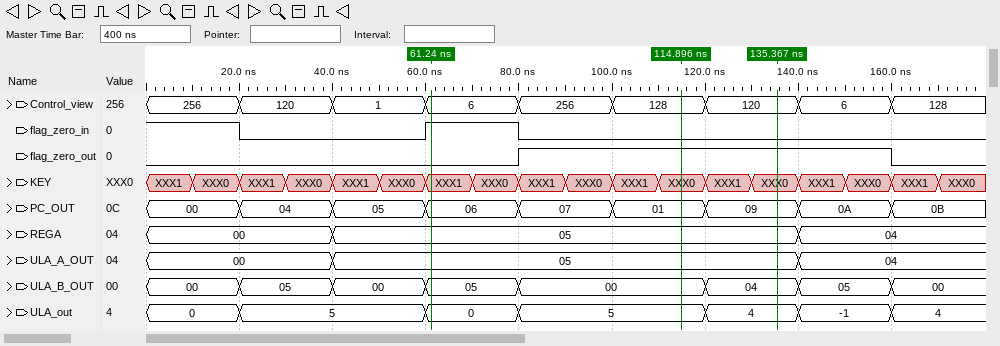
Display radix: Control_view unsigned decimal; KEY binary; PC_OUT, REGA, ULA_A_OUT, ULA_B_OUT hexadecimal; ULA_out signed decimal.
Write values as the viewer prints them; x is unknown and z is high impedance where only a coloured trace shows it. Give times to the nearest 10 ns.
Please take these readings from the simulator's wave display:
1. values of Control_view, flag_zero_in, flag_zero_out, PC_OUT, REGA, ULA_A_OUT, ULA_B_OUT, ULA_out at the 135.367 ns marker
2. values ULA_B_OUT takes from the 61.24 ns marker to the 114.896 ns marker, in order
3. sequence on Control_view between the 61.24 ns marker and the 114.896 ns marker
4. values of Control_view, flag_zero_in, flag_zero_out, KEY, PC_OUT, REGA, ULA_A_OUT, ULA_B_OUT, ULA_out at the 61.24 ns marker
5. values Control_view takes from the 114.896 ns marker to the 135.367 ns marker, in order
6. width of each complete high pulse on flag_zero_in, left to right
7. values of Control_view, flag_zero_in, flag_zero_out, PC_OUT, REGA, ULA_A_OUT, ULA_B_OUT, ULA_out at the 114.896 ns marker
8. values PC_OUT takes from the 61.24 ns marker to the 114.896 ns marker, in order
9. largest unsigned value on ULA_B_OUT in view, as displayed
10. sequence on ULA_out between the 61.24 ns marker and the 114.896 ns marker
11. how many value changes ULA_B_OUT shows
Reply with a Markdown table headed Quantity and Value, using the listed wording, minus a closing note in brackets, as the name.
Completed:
| Quantity | Value |
|---|---|
| values of Control_view, flag_zero_in, flag_zero_out, PC_OUT, REGA, ULA_A_OUT, ULA_B_OUT, ULA_out at the 135.367 ns marker | Control_view=120, flag_zero_in=0, flag_zero_out=1, PC_OUT=09, REGA=05, ULA_A_OUT=05, ULA_B_OUT=04, ULA_out=4 |
| values ULA_B_OUT takes from the 61.24 ns marker to the 114.896 ns marker, in order | 05, 00 |
| sequence on Control_view between the 61.24 ns marker and the 114.896 ns marker | 6, 256, 128 |
| values of Control_view, flag_zero_in, flag_zero_out, KEY, PC_OUT, REGA, ULA_A_OUT, ULA_B_OUT, ULA_out at the 61.24 ns marker | Control_view=6, flag_zero_in=1, flag_zero_out=0, KEY=XXX1, PC_OUT=06, REGA=05, ULA_A_OUT=05, ULA_B_OUT=05, ULA_out=0 |
| values Control_view takes from the 114.896 ns marker to the 135.367 ns marker, in order | 128, 120 |
| width of each complete high pulse on flag_zero_in, left to right | 20 ns |
| values of Control_view, flag_zero_in, flag_zero_out, PC_OUT, REGA, ULA_A_OUT, ULA_B_OUT, ULA_out at the 114.896 ns marker | Control_view=128, flag_zero_in=0, flag_zero_out=1, PC_OUT=01, REGA=05, ULA_A_OUT=05, ULA_B_OUT=00, ULA_out=5 |
| values PC_OUT takes from the 61.24 ns marker to the 114.896 ns marker, in order | 06, 07, 01 |
| largest unsigned value on ULA_B_OUT in view, as displayed | 05 |
| sequence on ULA_out between the 61.24 ns marker and the 114.896 ns marker | 0, 5 |
| how many value changes ULA_B_OUT shows | 7 |
